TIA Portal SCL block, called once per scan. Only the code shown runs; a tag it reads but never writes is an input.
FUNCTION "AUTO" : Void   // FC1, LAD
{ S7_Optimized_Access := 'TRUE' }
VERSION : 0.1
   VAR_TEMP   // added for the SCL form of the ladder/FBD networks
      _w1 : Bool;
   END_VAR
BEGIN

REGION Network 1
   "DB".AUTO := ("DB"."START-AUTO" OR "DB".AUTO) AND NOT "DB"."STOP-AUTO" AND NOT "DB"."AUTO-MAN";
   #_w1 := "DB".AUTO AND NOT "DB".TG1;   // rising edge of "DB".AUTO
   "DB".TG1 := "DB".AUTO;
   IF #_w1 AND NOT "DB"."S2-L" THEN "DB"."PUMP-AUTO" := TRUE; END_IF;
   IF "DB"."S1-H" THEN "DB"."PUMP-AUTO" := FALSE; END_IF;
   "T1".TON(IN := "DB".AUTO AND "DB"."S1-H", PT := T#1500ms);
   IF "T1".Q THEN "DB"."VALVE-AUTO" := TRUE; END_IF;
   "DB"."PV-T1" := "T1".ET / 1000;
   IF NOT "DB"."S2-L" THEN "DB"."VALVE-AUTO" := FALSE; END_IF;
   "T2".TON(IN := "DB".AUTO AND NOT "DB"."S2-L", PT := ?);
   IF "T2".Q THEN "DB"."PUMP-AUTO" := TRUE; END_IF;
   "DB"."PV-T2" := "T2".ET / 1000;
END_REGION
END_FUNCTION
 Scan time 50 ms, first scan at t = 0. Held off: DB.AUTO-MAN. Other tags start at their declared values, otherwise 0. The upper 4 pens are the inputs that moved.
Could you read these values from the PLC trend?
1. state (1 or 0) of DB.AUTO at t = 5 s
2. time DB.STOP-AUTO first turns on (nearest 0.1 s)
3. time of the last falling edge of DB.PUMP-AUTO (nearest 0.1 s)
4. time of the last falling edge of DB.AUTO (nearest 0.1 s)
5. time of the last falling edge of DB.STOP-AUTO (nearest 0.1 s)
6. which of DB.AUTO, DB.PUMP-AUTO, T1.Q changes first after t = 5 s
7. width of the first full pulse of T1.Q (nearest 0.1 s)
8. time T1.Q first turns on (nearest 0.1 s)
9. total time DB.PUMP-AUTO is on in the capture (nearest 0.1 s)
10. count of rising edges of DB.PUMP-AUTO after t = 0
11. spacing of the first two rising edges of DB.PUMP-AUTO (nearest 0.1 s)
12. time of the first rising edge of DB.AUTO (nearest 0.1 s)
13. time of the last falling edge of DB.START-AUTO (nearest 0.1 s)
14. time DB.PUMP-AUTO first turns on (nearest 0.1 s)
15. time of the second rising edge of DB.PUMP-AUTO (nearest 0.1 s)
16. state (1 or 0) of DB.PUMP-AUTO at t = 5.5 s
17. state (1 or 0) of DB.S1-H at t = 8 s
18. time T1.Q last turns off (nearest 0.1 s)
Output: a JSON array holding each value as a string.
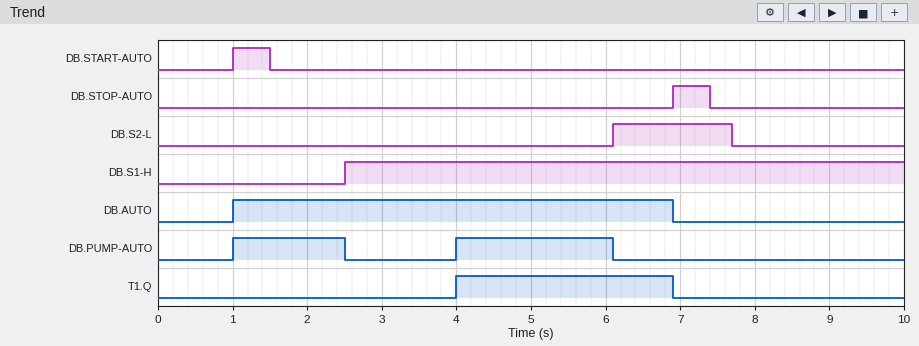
["1", "6.9 s", "6.1 s", "6.9 s", "7.4 s", "DB.PUMP-AUTO", "2.9 s", "4.0 s", "3.6 s", "2", "3.0 s", "1.0 s", "1.5 s", "1.0 s", "4.0 s", "1", "1", "6.9 s"]
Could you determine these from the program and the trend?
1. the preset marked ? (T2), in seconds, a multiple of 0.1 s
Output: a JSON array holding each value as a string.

["3.0 s"]
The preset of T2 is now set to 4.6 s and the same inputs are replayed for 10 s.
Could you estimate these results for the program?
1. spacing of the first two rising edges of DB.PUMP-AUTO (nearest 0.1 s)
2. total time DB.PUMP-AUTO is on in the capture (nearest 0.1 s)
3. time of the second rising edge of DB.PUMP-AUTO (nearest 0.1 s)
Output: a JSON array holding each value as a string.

["4.6 s", "2.0 s", "5.6 s"]
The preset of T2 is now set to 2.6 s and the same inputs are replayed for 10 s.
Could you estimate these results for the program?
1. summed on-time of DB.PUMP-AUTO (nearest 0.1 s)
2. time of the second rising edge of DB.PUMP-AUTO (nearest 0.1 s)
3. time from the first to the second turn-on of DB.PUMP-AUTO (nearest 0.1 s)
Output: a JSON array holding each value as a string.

["4.0 s", "3.6 s", "2.6 s"]
